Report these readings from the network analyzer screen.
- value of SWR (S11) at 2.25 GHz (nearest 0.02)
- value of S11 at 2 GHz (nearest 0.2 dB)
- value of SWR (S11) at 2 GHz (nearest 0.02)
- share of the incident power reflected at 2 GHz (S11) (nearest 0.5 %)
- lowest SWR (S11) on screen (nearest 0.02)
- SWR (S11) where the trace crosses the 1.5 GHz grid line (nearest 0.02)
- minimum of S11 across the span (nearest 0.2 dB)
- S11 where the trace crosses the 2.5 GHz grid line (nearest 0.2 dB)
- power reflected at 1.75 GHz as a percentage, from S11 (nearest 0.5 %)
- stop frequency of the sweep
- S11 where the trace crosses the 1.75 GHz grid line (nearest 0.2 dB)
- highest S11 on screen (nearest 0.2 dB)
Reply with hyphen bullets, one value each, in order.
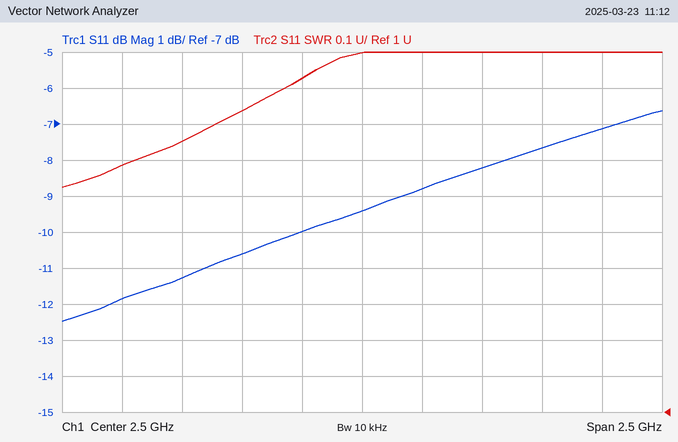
- 1.92
- -10.6 dB
- 1.84
- 8.5 %
- 1.62
- 1.68
- -12.4 dB
- -9.4 dB
- 7.5 %
- 3.75 GHz
- -11.2 dB
- -6.6 dB
